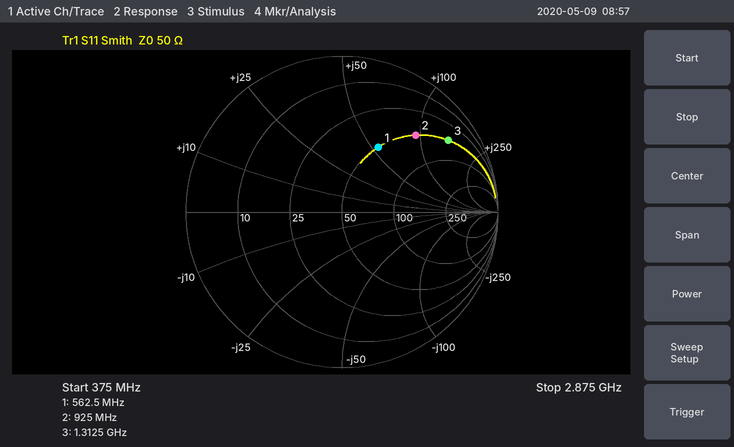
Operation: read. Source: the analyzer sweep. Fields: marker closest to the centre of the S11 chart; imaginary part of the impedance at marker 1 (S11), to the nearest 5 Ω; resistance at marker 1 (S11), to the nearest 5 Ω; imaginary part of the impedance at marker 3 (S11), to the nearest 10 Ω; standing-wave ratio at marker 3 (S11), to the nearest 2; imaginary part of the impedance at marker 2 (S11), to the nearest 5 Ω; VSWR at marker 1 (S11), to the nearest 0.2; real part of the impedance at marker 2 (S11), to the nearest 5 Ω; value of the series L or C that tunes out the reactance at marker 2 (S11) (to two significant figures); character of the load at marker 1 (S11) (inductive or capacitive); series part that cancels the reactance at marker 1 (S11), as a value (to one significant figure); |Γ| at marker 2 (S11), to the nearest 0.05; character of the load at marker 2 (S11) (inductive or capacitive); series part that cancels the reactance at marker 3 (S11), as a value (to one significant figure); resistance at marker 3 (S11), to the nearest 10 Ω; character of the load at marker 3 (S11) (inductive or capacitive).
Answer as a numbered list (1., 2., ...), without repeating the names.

1. marker 1
2. +55 Ω
3. 50 Ω
4. +150 Ω
5. 10
6. +95 Ω
7. 2.8
8. 50 Ω
9. 1.8 pF
10. inductive
11. 5 pF
12. 0.70
13. inductive
14. 800 fF
15. 50 Ω
16. inductive
